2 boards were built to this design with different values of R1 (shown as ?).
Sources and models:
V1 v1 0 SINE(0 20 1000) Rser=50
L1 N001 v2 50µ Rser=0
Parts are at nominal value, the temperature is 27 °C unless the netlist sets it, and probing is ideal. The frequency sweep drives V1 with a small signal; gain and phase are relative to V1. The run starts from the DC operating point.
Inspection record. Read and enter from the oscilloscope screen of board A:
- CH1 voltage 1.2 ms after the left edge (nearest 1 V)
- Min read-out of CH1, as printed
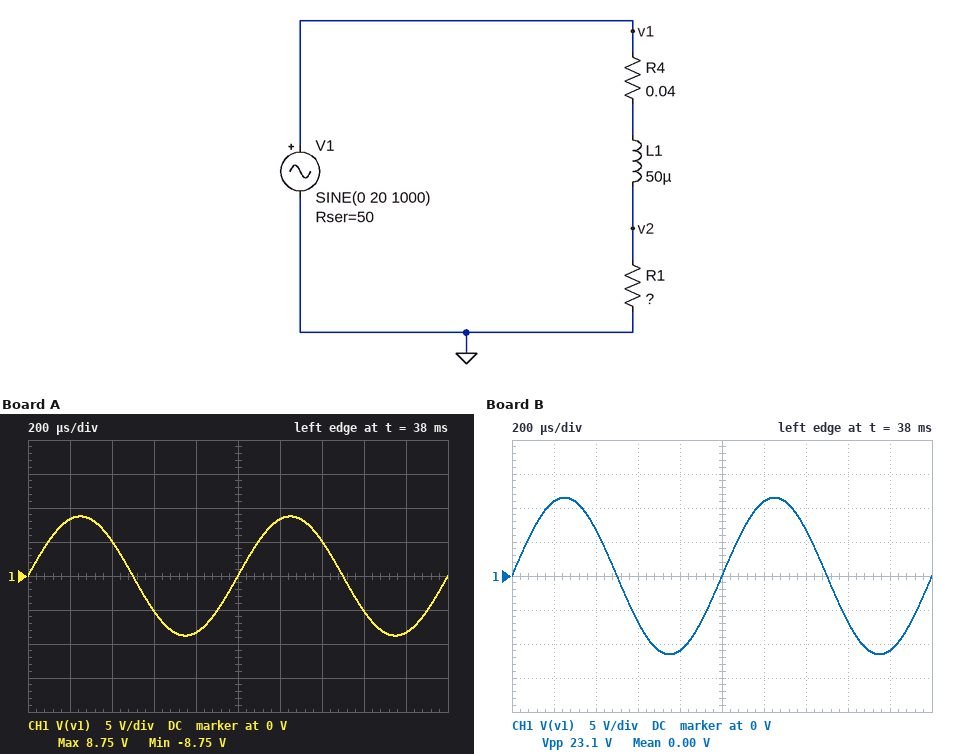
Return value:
8 V
-8.75 V
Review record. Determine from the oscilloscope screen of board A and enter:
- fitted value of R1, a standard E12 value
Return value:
39 Ω
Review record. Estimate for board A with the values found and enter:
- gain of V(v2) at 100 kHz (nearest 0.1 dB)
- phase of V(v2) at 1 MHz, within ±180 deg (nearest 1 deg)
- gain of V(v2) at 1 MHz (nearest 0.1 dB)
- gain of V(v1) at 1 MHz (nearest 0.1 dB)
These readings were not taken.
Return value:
-7.7 dB
-74 deg
-18.5 dB
-0.3 dB
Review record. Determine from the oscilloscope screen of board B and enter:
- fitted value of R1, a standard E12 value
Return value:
68 Ω
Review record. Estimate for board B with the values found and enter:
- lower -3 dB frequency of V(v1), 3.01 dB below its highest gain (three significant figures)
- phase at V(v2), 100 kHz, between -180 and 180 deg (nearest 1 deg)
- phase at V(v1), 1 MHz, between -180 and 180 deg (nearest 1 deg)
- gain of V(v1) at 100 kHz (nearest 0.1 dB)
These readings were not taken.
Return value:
218 kHz
-15 deg
8 deg
-4.2 dB
